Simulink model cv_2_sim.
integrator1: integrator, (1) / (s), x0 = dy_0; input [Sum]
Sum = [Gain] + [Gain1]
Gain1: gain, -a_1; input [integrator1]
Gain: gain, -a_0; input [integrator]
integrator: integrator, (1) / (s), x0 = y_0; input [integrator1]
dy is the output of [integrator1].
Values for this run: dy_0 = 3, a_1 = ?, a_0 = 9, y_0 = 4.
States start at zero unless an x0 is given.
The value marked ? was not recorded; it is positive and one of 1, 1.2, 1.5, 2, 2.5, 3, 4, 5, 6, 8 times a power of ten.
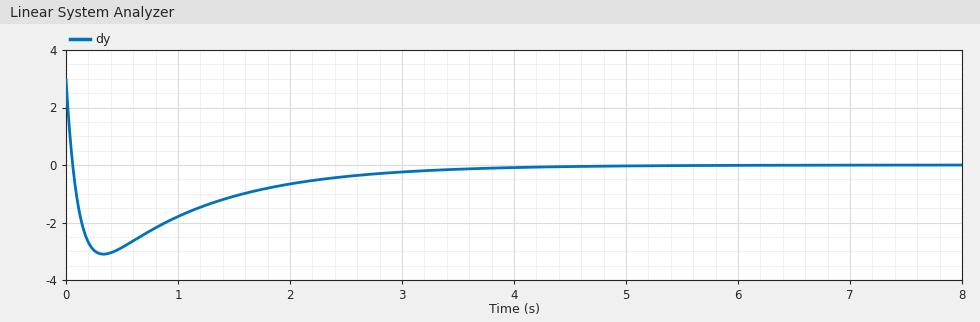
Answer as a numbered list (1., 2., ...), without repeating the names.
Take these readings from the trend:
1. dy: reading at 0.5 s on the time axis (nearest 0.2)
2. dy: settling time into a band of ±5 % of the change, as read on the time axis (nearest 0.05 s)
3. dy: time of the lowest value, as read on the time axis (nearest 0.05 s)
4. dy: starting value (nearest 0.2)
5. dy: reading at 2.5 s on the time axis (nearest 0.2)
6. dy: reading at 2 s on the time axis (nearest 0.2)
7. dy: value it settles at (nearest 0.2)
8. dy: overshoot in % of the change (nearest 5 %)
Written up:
1. -2.8
2. 3.50 s
3. 0.35 s
4. 3.0
5. -0.4
6. -0.6
7. 0.0
8. 105 %
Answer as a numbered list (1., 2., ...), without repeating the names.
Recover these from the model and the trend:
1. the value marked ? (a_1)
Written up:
1. 10
